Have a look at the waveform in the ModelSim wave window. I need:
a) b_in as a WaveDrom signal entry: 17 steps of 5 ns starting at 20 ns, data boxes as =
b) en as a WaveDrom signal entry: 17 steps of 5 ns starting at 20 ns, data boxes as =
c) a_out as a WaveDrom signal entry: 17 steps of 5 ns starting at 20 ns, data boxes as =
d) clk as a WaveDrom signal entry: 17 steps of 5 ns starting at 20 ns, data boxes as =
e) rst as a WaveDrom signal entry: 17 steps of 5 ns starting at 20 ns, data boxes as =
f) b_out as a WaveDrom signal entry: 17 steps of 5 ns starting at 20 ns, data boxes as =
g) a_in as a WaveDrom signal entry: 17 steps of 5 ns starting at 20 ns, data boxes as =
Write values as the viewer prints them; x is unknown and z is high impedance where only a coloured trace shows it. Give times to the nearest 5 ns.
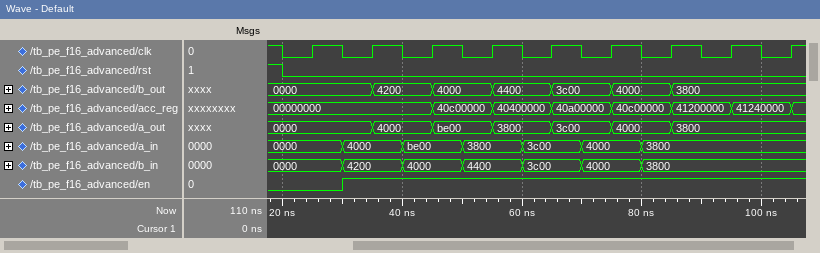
{name: 'b_in', wave: '=.=.=.=.=.=.=....', data: '0000 4200 4000 4400 3c00 4000 3800'}
{name: 'en', wave: '0.1..............'}
{name: 'a_out', wave: '=..=.=.=.=.=.=...', data: '0000 4000 be00 3800 3c00 4000 3800'}
{name: 'clk', wave: '01010101010101010'}
{name: 'rst', wave: '0................'}
{name: 'b_out', wave: '=..=.=.=.=.=.=...', data: '0000 4200 4000 4400 3c00 4000 3800'}
{name: 'a_in', wave: '=.=.=.=.=.=.=....', data: '0000 4000 be00 3800 3c00 4000 3800'}
